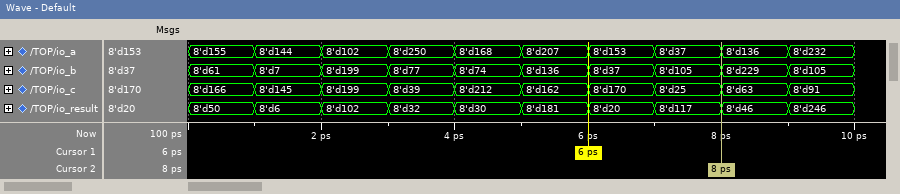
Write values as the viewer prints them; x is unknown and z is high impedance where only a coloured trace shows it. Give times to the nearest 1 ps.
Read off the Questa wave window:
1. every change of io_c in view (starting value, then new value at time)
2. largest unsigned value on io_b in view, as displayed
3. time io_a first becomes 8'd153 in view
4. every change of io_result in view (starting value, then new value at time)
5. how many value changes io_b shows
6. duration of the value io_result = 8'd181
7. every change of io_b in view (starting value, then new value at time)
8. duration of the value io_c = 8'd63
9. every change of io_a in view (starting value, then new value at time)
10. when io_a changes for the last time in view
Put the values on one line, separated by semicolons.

8'd166, 8'd145 at 1 ps, 8'd199 at 2 ps, 8'd39 at 3 ps, 8'd212 at 4 ps, 8'd162 at 5 ps, 8'd170 at 6 ps, 8'd25 at 7 ps, 8'd63 at 8 ps, 8'd91 at 9 ps; 8'd229; 6 ps; 8'd50, 8'd6 at 1 ps, 8'd102 at 2 ps, 8'd32 at 3 ps, 8'd30 at 4 ps, 8'd181 at 5 ps, 8'd20 at 6 ps, 8'd117 at 7 ps, 8'd46 at 8 ps, 8'd246 at 9 ps; 9; 1 ps; 8'd61, 8'd7 at 1 ps, 8'd199 at 2 ps, 8'd77 at 3 ps, 8'd74 at 4 ps, 8'd136 at 5 ps, 8'd37 at 6 ps, 8'd105 at 7 ps, 8'd229 at 8 ps, 8'd105 at 9 ps; 1 ps; 8'd155, 8'd144 at 1 ps, 8'd102 at 2 ps, 8'd250 at 3 ps, 8'd168 at 4 ps, 8'd207 at 5 ps, 8'd153 at 6 ps, 8'd37 at 7 ps, 8'd136 at 8 ps, 8'd232 at 9 ps; 9 ps
